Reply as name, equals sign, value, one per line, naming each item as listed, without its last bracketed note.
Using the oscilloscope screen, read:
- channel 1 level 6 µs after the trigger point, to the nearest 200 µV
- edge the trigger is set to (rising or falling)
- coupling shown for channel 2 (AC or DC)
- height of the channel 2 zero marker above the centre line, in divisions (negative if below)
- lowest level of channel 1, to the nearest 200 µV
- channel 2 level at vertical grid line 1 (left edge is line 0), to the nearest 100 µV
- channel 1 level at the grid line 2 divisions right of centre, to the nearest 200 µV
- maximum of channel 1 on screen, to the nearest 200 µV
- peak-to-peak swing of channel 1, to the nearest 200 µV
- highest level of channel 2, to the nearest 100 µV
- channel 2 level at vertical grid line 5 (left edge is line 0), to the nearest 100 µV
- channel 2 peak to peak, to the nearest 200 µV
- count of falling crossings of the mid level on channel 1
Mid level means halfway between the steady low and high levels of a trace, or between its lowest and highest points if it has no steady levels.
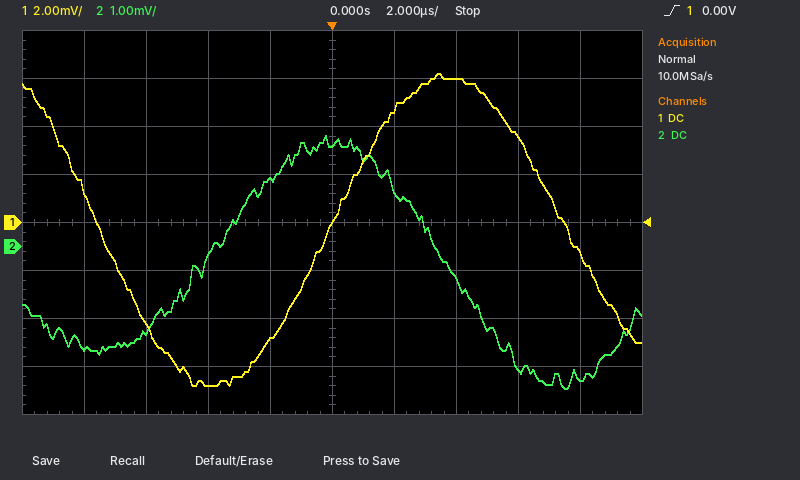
channel 1 level 6 µs after the trigger point, to the nearest 200 µV = 3.6 mV
edge the trigger is set to = rising
coupling shown for channel 2 = DC
height of the channel 2 zero marker above the centre line, in divisions = -0.5 div
lowest level of channel 1, to the nearest 200 µV = -6.8 mV
channel 2 level at vertical grid line 1 (left edge is line 0), to the nearest 100 µV = -2.1 mV
channel 1 level at the grid line 2 divisions right of centre, to the nearest 200 µV = 6.0 mV
maximum of channel 1 on screen, to the nearest 200 µV = 6.2 mV
peak-to-peak swing of channel 1, to the nearest 200 µV = 13.0 mV
highest level of channel 2, to the nearest 100 µV = 2.3 mV
channel 2 level at vertical grid line 5 (left edge is line 0), to the nearest 100 µV = 2.1 mV
channel 2 peak to peak, to the nearest 200 µV = 5.2 mV
count of falling crossings of the mid level on channel 1 = 2
